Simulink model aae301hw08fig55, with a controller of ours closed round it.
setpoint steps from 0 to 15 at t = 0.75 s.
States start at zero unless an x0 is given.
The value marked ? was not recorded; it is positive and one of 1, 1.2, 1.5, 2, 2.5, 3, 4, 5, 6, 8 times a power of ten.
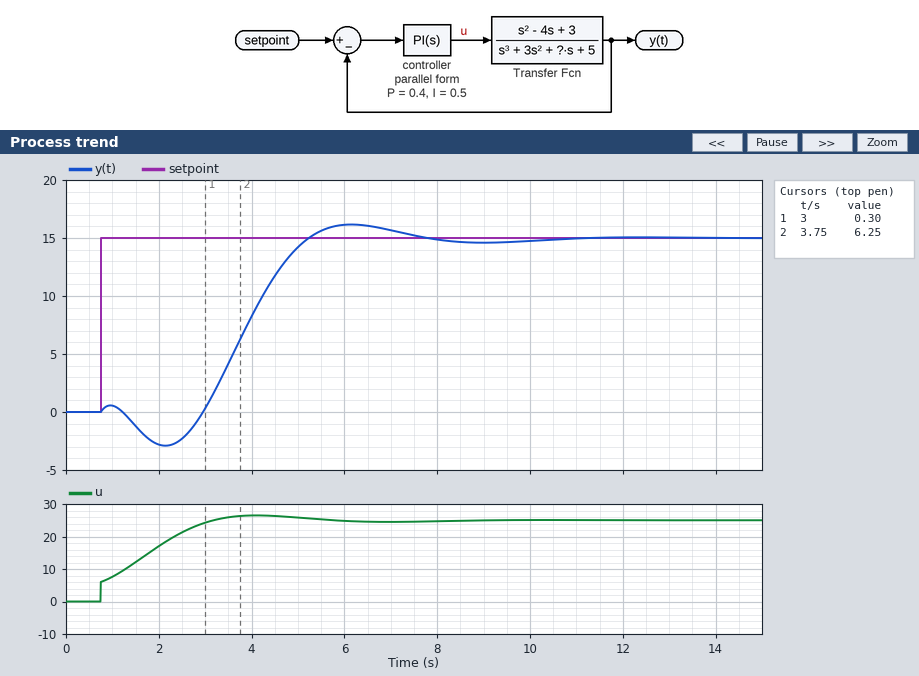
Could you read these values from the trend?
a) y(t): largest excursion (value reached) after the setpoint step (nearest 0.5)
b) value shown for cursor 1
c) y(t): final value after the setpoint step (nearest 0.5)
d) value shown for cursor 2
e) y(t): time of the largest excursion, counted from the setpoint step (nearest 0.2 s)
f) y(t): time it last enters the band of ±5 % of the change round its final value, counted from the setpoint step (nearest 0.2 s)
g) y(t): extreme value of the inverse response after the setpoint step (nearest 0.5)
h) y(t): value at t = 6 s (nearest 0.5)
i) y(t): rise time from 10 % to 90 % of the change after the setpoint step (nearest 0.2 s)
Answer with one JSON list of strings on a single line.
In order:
["16.0", "0.30", "15.0", "6.25", "5.4 s", "6.2 s", "-3.0", "16.0", "1.6 s"]
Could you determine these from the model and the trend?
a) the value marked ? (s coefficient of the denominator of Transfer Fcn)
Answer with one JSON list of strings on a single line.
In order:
["6"]
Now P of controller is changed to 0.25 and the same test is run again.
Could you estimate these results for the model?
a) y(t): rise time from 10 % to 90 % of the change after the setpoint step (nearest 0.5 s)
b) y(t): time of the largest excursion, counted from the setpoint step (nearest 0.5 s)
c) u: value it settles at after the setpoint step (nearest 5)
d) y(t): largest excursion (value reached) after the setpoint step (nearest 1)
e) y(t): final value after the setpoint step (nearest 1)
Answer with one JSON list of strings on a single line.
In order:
["2.0 s", "6.5 s", "25", "17", "15"]
